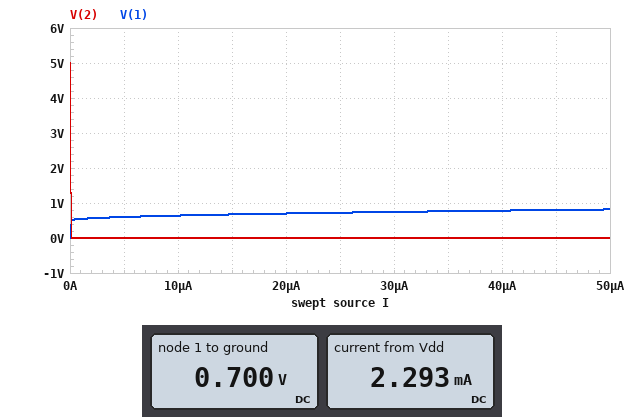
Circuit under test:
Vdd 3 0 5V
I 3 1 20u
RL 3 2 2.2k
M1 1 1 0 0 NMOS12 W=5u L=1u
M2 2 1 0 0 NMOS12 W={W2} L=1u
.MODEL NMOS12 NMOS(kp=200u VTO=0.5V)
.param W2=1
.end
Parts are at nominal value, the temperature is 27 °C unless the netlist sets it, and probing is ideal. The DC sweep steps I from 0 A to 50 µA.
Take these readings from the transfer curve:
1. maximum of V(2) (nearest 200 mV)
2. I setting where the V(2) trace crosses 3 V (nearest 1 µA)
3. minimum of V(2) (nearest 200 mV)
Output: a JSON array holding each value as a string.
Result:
["5.0 V", "0 A", "0 V"]
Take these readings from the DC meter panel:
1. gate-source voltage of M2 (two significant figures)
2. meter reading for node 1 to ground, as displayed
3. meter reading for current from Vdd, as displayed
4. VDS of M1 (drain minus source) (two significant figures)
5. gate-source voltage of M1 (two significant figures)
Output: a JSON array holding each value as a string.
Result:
["700 mV", "0.700 V", "2.293 mA", "700 mV", "700 mV"]
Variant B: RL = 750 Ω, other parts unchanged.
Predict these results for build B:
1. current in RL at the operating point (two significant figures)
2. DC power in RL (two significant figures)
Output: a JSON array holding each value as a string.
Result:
["6.7 mA", "33 mW"]
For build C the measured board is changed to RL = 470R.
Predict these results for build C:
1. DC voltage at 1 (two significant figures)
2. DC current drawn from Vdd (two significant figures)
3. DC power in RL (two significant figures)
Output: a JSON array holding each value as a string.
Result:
["700 mV", "11 mA", "53 mW"]
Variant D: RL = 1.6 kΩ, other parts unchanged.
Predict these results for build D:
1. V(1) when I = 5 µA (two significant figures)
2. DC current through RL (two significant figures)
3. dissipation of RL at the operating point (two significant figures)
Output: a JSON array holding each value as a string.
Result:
["600 mV", "3.1 mA", "16 mW"]
